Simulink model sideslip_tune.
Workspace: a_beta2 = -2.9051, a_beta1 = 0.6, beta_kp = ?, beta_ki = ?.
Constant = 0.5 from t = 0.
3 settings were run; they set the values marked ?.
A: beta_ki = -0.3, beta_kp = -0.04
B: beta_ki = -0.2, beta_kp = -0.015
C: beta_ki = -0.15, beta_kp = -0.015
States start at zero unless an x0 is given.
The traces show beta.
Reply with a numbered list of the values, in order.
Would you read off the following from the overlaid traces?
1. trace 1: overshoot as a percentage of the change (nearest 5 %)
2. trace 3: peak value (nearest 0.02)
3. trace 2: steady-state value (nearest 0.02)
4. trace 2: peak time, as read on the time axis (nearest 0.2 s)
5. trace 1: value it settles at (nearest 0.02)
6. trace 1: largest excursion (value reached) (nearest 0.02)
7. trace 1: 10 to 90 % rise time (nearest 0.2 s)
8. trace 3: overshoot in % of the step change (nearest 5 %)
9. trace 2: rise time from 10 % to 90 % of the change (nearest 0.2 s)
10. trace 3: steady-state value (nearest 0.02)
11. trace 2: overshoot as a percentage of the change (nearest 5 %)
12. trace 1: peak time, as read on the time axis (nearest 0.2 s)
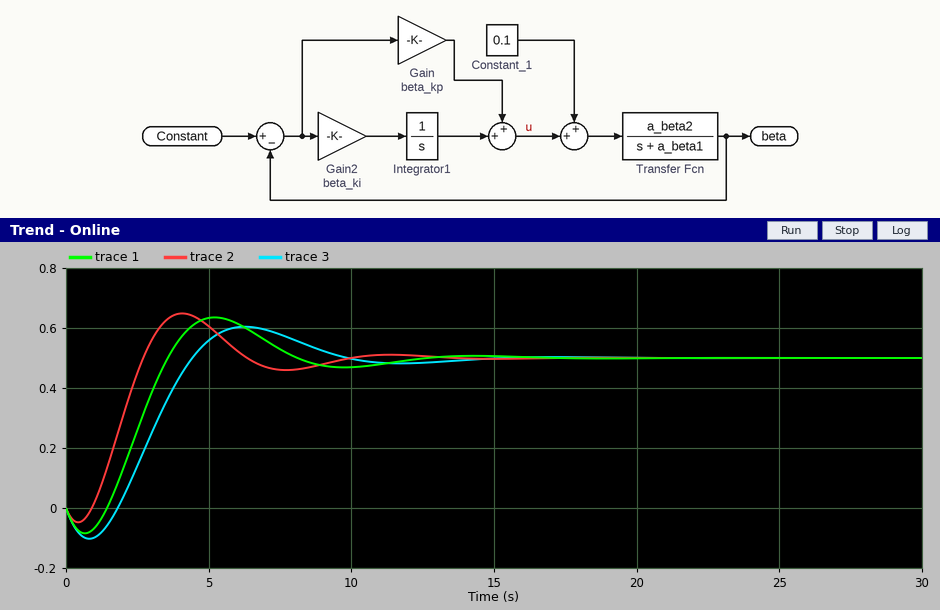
1. 25 %
2. 0.60
3. 0.50
4. 4.0 s
5. 0.50
6. 0.64
7. 1.6 s
8. 20 %
9. 1.4 s
10. 0.50
11. 30 %
12. 5.2 s
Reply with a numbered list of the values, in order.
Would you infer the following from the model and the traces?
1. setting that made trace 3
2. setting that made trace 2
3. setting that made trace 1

1. C
2. A
3. B
